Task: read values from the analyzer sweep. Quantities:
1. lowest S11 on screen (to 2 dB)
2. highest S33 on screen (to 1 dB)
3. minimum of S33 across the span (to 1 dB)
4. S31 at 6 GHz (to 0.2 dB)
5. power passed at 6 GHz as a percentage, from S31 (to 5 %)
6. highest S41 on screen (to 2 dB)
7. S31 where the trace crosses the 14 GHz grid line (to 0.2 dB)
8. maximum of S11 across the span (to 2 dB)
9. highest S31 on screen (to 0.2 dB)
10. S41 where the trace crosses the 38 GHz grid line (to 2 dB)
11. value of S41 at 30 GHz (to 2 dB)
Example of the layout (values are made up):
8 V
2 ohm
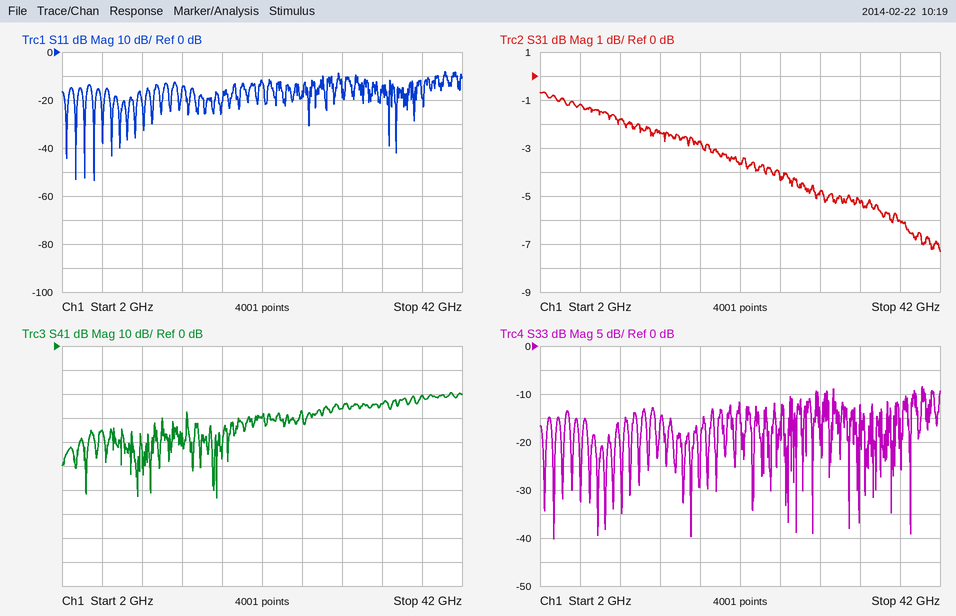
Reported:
-54 dB
-8 dB
-40 dB
-1.2 dB
75 %
-20 dB
-2.4 dB
-8 dB
-0.6 dB
-20 dB
-26 dB
